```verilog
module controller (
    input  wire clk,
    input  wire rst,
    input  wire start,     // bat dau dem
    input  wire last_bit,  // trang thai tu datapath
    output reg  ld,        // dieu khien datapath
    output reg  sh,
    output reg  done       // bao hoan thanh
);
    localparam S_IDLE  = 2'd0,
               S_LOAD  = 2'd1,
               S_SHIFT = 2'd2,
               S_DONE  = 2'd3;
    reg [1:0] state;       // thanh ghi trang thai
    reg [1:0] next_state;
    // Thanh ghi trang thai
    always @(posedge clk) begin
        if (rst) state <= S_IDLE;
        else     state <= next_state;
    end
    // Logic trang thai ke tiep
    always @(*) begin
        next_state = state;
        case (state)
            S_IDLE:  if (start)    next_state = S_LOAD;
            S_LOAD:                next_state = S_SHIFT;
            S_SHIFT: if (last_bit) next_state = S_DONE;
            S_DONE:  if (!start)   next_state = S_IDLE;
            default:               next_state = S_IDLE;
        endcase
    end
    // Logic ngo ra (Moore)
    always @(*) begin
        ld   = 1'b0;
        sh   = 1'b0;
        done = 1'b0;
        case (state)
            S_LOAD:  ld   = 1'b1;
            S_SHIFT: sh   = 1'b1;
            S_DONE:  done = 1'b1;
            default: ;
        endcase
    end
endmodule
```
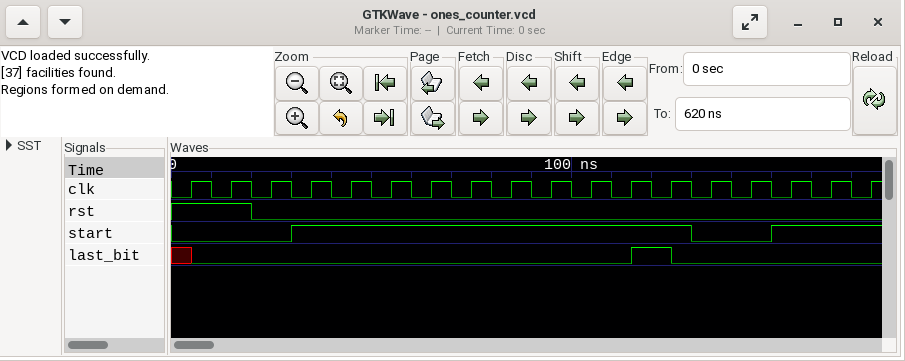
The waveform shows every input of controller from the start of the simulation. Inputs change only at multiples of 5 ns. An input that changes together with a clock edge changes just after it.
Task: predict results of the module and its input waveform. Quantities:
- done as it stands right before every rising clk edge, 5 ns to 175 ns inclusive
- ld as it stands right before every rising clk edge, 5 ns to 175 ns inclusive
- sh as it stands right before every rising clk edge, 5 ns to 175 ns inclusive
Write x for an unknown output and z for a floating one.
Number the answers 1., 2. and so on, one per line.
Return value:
1. x 0 0 0 0 0 0 0 0 0 0 0 0 1 0 0 0 0
2. x 0 0 0 1 0 0 0 0 0 0 0 0 0 0 0 1 0
3. x 0 0 0 0 1 1 1 1 1 1 1 1 0 0 0 0 1
